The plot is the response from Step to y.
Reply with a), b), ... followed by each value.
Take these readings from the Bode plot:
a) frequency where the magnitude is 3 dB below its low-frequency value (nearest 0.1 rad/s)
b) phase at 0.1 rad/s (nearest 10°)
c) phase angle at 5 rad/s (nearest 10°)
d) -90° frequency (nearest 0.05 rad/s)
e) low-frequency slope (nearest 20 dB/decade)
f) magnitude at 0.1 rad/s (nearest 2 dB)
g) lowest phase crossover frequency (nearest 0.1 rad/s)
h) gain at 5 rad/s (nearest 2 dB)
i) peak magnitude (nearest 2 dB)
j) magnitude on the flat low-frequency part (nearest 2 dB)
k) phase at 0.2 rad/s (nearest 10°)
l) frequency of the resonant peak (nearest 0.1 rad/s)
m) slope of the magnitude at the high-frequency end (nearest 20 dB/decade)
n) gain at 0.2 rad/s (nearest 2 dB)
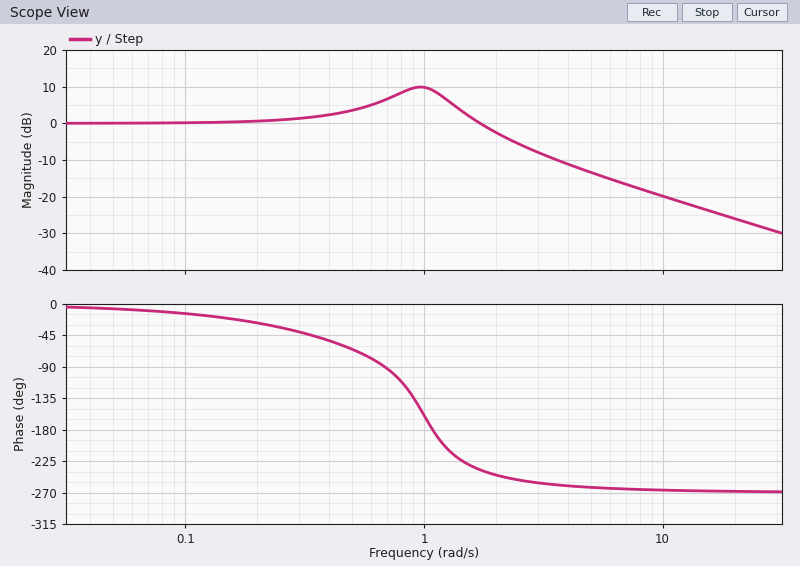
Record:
a) 2.1 rad/s
b) -10°
c) -260°
d) 0.70 rad/s
e) 0 dB/decade
f) 0 dB
g) 1.1 rad/s
h) -14 dB
i) 10 dB
j) 0 dB
k) -30°
l) 1.0 rad/s
m) -20 dB/decade
n) 0 dB
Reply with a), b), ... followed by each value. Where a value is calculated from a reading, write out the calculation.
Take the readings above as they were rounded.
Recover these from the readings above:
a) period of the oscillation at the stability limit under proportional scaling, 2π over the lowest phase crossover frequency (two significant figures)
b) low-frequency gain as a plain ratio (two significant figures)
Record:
a) 2π / 1.1 = 5.7 s
b) 10^(0 / 20) = 1.0
